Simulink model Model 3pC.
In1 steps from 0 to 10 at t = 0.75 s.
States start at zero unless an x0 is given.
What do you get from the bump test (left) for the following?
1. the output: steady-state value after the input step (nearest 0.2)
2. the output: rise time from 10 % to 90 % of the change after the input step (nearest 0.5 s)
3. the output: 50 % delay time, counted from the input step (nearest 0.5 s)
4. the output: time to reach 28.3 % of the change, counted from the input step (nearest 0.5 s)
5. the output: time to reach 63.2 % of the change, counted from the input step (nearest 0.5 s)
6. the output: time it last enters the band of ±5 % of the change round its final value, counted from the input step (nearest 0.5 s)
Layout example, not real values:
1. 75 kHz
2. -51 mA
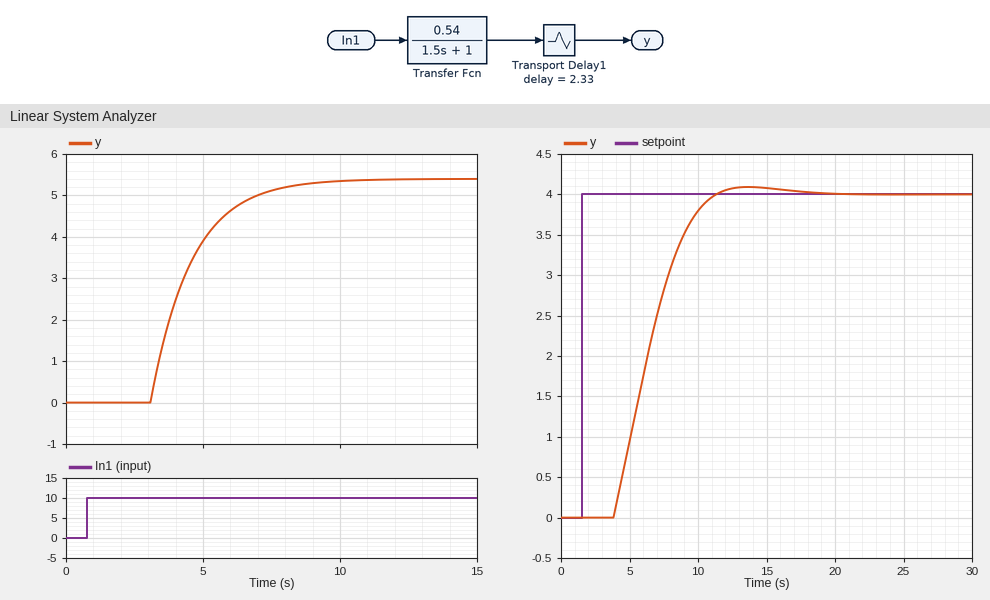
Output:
1. 5.4
2. 3.5 s
3. 3.5 s
4. 3.0 s
5. 4.0 s
6. 7.0 s
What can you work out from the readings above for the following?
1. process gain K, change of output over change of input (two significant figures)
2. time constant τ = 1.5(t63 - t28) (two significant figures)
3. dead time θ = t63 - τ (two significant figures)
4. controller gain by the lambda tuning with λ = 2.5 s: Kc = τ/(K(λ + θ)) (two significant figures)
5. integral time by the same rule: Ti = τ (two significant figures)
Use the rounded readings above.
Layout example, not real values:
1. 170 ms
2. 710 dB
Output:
1. 0.54
2. 1.5 s
3. 2.5 s
4. 0.56
5. 1.5 s
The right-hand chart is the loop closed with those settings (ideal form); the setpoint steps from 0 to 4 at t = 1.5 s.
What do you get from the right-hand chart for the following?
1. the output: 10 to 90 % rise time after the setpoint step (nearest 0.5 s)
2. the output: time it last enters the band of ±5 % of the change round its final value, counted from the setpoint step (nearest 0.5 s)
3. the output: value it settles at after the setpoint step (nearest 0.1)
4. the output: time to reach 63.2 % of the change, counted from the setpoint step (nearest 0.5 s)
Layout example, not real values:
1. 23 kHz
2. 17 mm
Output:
1. 5.0 s
2. 8.5 s
3. 4.0
4. 5.5 s
